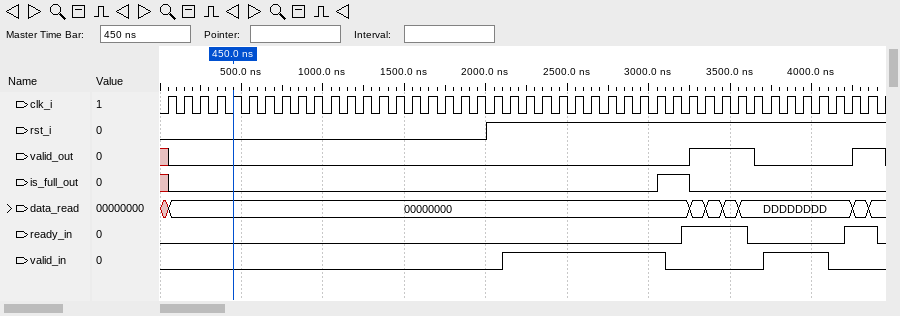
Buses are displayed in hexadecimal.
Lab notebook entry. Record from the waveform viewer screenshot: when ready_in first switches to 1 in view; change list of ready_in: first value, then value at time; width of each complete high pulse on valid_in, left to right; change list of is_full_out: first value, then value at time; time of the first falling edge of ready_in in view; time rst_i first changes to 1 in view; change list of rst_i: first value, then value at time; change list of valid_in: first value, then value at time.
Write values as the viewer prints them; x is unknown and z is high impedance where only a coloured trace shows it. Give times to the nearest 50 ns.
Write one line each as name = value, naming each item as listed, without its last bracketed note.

when ready_in first switches to 1 in view = 3200 ns
change list of ready_in: first value, then value at time = 0, 1 at 3200 ns, 0 at 3600 ns, 1 at 4200 ns, 0 at 4400 ns
width of each complete high pulse on valid_in, left to right = 1000 ns, 400 ns
change list of is_full_out: first value, then value at time = x, 0 at 50 ns, 1 at 3050 ns, 0 at 3250 ns
time of the first falling edge of ready_in in view = 3600 ns
time rst_i first changes to 1 in view = 2000 ns
change list of rst_i: first value, then value at time = 0, 1 at 2000 ns
change list of valid_in: first value, then value at time = 0, 1 at 2100 ns, 0 at 3100 ns, 1 at 3700 ns, 0 at 4100 ns
